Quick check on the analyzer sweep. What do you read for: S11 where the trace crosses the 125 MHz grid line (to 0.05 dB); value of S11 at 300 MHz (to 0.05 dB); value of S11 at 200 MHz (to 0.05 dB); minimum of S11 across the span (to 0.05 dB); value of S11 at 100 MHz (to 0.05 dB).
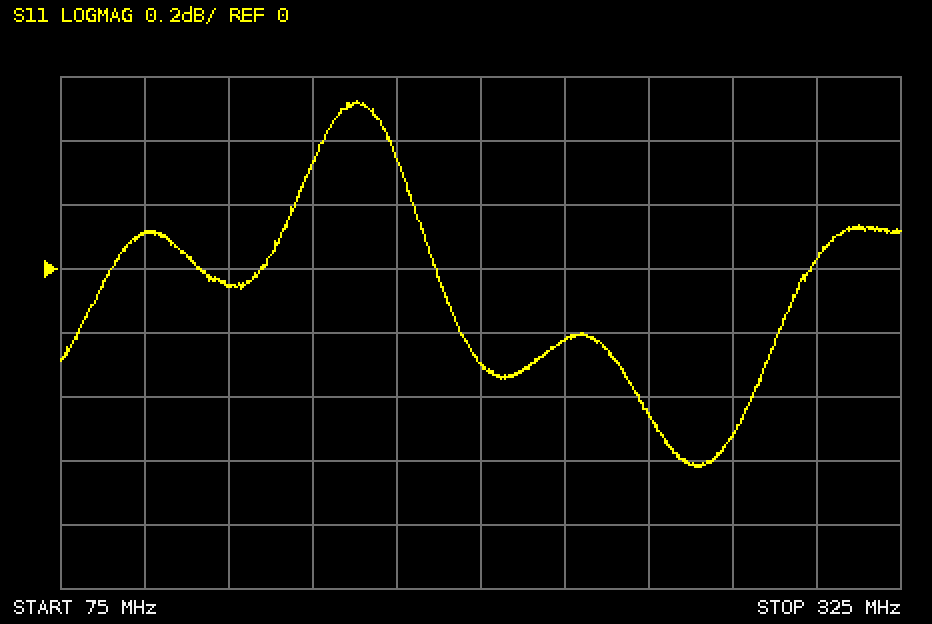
-0.05 dB
0.05 dB
-0.30 dB
-0.60 dB
0.10 dB
